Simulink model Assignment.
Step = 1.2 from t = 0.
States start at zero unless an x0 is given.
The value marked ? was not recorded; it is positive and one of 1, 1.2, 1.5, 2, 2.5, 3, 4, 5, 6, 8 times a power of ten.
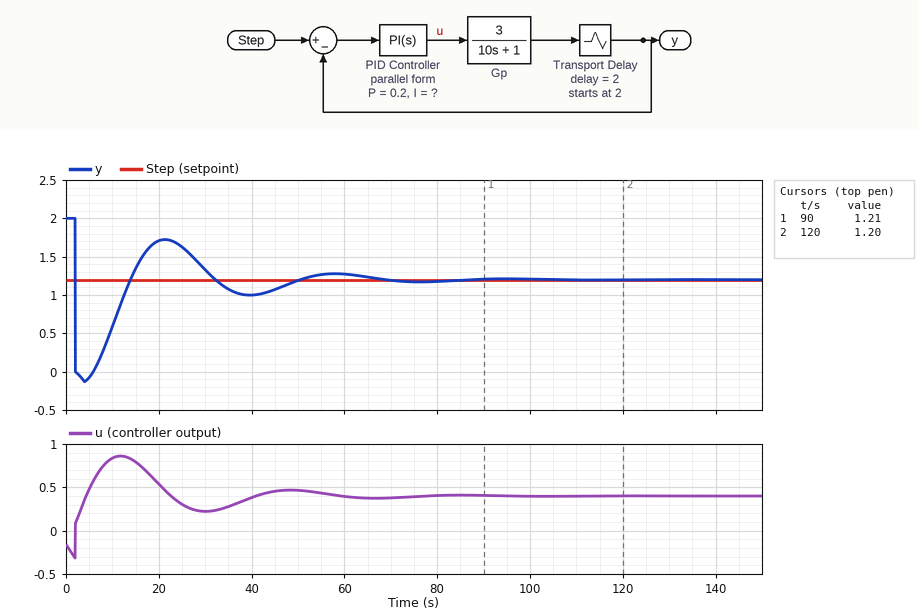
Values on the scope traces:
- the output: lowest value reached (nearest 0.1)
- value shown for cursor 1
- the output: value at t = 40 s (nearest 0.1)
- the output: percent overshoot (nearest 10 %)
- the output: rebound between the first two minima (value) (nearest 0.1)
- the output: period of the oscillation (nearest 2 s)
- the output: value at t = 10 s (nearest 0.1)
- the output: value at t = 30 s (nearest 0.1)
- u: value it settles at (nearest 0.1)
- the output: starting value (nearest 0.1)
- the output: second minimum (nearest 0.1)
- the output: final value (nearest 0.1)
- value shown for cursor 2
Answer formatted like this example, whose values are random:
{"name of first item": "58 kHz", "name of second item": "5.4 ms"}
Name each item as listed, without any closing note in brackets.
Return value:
{"the output: lowest value reached": "-0.1", "value shown for cursor 1": "1.21", "the output: value at t = 40 s": "1.0", "the output: percent overshoot": "170 %", "the output: rebound between the first two minima (value)": "1.7", "the output: period of the oscillation": "36 s", "the output: value at t = 10 s": "0.6", "the output: value at t = 30 s": "1.3", "u: value it settles at": "0.4", "the output: starting value": "2.0", "the output: second minimum": "1.0", "the output: final value": "1.2", "value shown for cursor 2": "1.20"}
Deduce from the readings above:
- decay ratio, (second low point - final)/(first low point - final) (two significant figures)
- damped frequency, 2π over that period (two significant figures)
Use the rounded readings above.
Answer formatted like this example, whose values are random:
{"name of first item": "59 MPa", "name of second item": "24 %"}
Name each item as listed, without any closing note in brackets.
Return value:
{"decay ratio, (second low point - final)/(first low point - final)": "0.15", "damped frequency, 2π over that period": "0.17 rad/s"}
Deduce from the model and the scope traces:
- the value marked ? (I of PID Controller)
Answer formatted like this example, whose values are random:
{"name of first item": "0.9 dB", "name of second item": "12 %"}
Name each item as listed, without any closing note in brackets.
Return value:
{"the value marked ?": "0.1"}
